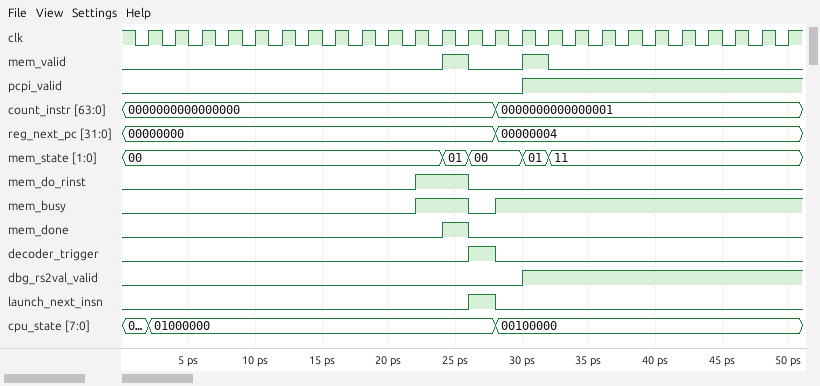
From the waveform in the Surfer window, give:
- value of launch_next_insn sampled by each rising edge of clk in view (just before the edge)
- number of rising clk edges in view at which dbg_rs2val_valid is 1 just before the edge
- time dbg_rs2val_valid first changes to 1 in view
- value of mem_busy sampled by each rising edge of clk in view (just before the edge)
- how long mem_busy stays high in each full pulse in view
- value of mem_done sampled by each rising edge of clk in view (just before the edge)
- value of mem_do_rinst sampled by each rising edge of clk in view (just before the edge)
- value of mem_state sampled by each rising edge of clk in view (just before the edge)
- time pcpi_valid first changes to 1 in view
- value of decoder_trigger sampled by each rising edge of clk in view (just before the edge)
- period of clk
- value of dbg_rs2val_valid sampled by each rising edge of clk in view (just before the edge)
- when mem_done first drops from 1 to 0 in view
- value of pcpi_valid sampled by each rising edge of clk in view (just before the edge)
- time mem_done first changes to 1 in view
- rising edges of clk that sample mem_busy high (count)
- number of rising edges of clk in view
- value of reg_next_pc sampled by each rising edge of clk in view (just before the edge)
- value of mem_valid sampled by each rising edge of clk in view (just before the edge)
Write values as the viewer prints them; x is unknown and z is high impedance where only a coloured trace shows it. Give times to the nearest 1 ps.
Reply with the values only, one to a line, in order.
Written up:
0 0 0 0 0 0 0 0 0 0 0 0 0 1 0 0 0 0 0 0 0 0 0 0 0
10
30 ps
0 0 0 0 0 0 0 0 0 0 0 1 1 0 1 1 1 1 1 1 1 1 1 1 1
4 ps
0 0 0 0 0 0 0 0 0 0 0 0 1 0 0 0 0 0 0 0 0 0 0 0 0
0 0 0 0 0 0 0 0 0 0 0 1 1 0 0 0 0 0 0 0 0 0 0 0 0
00, 00, 00, 00, 00, 00, 00, 00, 00, 00, 00, 00, 01, 00, 00, 01, 11, 11, 11, 11, 11, 11, 11, 11, 11
30 ps
0 0 0 0 0 0 0 0 0 0 0 0 0 1 0 0 0 0 0 0 0 0 0 0 0
2 ps
0 0 0 0 0 0 0 0 0 0 0 0 0 0 0 1 1 1 1 1 1 1 1 1 1
26 ps
0 0 0 0 0 0 0 0 0 0 0 0 0 0 0 1 1 1 1 1 1 1 1 1 1
24 ps
13
25
00000000, 00000000, 00000000, 00000000, 00000000, 00000000, 00000000, 00000000, 00000000, 00000000, 00000000, 00000000, 00000000, 00000000, 00000004, 00000004, 00000004, 00000004, 00000004, 00000004, 00000004, 00000004, 00000004, 00000004, 00000004
0 0 0 0 0 0 0 0 0 0 0 0 1 0 0 1 0 0 0 0 0 0 0 0 0
